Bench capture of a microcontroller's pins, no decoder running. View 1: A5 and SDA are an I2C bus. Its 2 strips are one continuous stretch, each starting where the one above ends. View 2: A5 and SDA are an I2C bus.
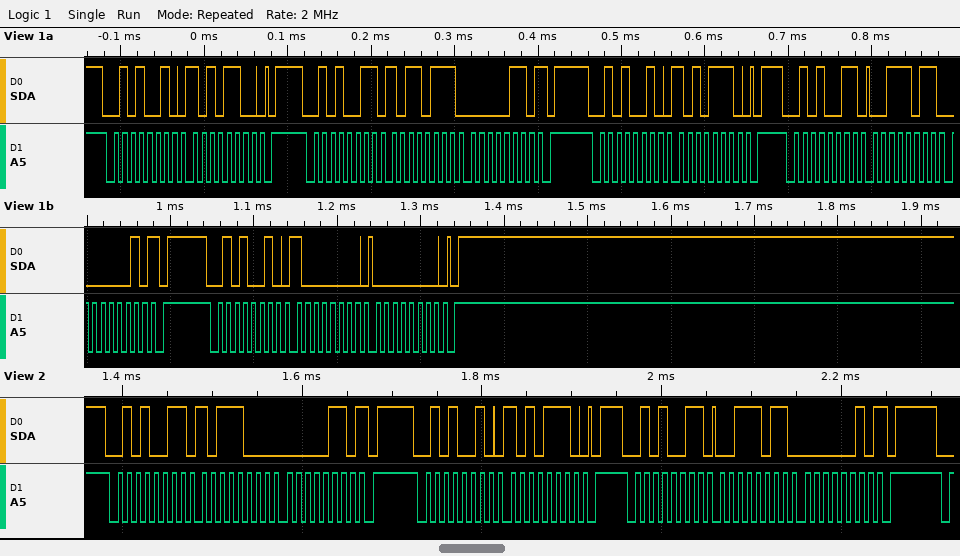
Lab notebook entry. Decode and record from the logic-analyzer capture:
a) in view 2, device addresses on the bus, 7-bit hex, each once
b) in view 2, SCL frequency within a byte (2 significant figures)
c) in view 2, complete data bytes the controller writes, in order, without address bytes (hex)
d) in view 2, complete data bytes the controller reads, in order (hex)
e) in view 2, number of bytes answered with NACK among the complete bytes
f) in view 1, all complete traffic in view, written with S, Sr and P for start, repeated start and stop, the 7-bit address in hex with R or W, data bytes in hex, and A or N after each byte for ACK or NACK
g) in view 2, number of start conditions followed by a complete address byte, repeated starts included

0x29
100 kHz
AE
B8 06 3B 02
2
S 29W A AC A P S 29R A B7 A 06 N P S 29W A AE A P S 29R A 3B A 02 N P S 29W A 80 A 00 A P
3
